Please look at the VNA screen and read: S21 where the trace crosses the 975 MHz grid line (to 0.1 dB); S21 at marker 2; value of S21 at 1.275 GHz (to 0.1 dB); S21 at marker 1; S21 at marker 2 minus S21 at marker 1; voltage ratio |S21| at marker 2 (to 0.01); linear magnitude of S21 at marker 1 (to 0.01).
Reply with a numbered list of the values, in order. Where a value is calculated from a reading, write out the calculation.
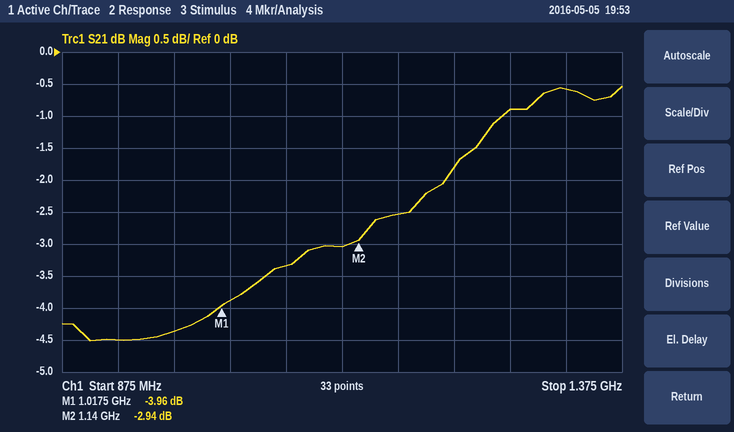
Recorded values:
1. -4.4 dB
2. -2.94 dB
3. -0.9 dB
4. -3.96 dB
5. -2.94 − (-3.96) = 1.02 dB
6. 10^(-2.94/20) ≈ 0.71
7. 10^(-3.96/20) ≈ 0.63
